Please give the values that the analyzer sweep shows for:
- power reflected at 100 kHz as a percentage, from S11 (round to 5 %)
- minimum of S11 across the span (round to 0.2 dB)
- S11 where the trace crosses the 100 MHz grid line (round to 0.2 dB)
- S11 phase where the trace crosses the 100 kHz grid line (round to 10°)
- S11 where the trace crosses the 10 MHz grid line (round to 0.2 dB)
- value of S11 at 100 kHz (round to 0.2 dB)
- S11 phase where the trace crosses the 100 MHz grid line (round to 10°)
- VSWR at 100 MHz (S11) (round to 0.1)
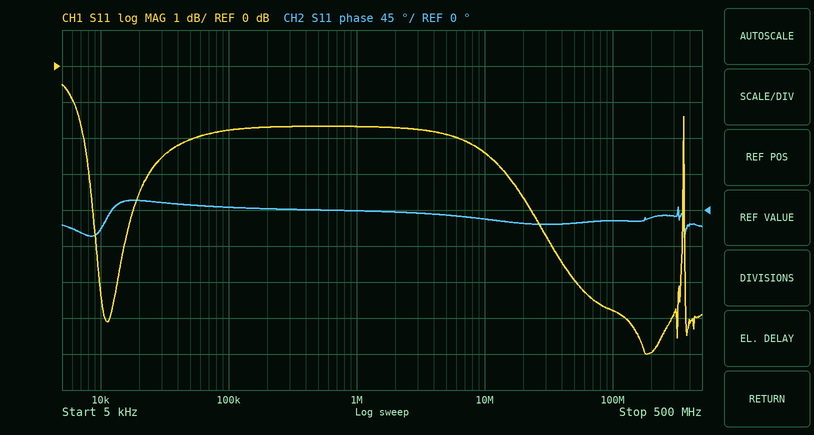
65 %
-8.0 dB
-6.8 dB
0°
-2.4 dB
-1.8 dB
-10°
2.7
